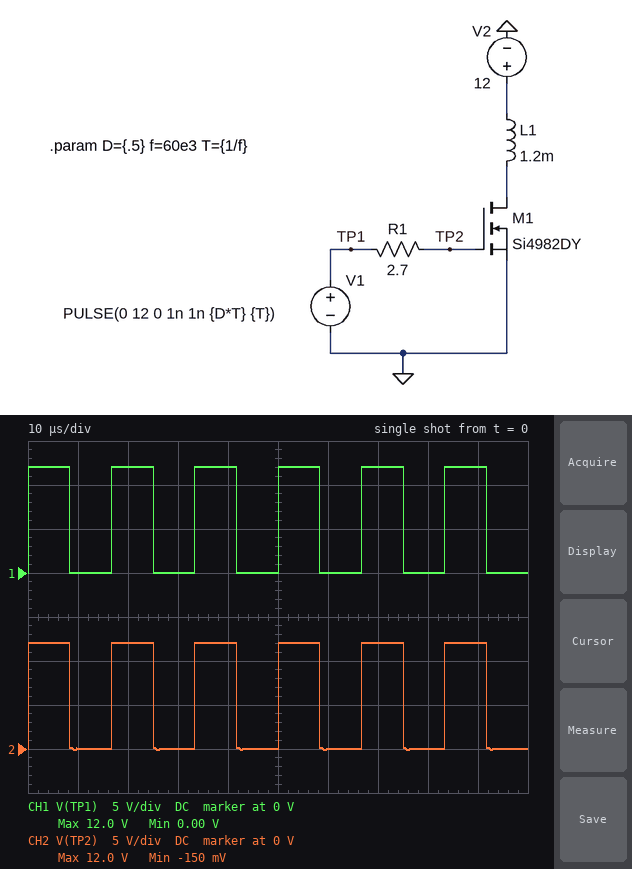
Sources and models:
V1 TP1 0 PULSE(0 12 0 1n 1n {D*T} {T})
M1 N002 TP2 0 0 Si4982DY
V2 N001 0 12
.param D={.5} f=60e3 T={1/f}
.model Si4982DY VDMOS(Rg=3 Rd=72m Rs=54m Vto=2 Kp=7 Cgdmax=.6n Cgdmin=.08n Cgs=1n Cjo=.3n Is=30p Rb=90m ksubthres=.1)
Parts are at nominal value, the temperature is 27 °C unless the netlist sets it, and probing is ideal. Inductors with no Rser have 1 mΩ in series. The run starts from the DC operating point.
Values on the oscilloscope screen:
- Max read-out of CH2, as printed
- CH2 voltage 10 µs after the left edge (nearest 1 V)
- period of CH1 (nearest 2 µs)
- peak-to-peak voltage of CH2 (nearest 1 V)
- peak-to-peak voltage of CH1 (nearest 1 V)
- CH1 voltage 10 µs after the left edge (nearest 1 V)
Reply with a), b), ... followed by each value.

a) 12.0 V
b) 0 V
c) 16 µs
d) 12 V
e) 12 V
f) 0 V
